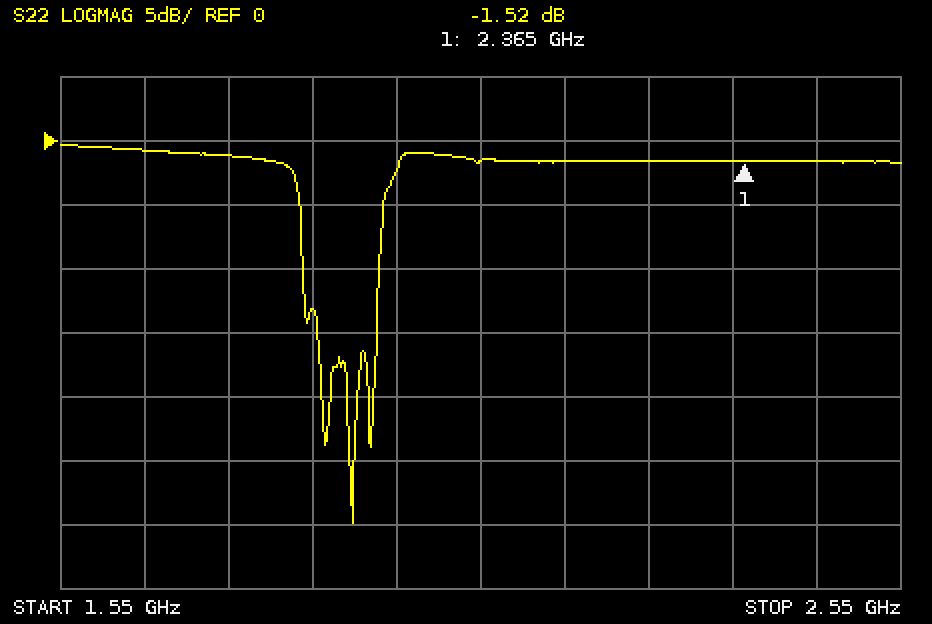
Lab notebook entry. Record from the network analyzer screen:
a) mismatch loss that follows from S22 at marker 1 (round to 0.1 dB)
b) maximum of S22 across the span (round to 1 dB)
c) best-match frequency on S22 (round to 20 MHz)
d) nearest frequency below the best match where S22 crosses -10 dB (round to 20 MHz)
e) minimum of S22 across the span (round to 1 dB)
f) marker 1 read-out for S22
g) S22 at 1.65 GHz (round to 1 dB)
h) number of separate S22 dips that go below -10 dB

5.3 dB
0 dB
1.90 GHz
1.84 GHz
-30 dB
-1.52 dB
-1 dB
3
